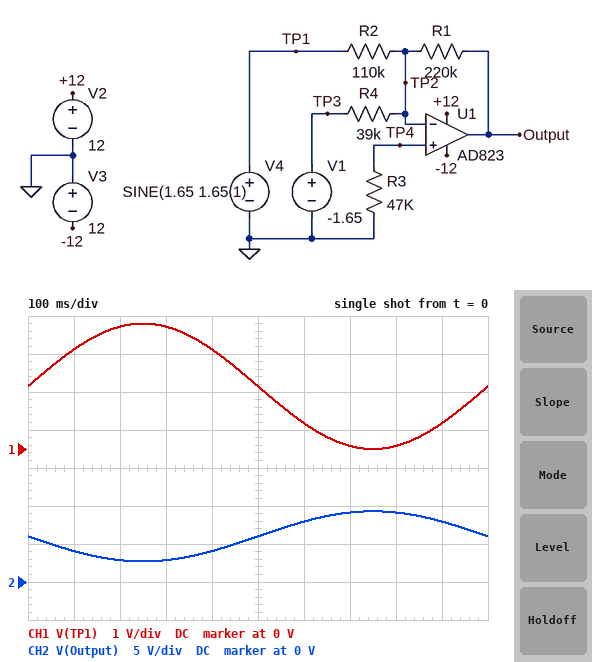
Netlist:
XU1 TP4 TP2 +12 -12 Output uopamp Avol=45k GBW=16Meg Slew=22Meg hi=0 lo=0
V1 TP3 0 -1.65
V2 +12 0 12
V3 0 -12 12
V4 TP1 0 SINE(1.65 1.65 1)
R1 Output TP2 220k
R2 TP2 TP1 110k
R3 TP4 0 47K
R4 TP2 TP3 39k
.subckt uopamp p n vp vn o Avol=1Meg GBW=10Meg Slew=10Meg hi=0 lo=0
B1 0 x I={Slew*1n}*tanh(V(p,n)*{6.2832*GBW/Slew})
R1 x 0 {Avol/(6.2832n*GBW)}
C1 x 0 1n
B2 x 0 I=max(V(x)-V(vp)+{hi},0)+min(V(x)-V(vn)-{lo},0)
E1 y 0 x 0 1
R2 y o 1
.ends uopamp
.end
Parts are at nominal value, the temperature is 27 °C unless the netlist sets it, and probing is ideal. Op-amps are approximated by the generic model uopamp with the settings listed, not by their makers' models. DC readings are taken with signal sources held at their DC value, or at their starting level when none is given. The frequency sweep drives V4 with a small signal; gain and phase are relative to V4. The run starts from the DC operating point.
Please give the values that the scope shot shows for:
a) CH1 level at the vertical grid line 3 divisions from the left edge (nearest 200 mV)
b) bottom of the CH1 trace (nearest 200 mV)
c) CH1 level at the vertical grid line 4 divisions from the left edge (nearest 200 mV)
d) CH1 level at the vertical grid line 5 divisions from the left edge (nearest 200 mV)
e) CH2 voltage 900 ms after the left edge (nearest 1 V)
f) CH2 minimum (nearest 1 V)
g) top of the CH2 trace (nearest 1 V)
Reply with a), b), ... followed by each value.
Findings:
a) 3.2 V
b) 0 V
c) 2.6 V
d) 1.6 V
e) 8 V
f) 3 V
g) 9 V
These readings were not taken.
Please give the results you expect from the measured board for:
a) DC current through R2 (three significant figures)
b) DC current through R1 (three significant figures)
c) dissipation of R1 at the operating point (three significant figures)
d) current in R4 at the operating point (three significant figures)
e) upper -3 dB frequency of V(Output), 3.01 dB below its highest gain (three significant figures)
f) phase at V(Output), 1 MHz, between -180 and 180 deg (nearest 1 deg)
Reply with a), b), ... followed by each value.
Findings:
a) 15.0 µA
b) 27.3 µA
c) 164 µW
d) 42.3 µA
e) 1.85 MHz
f) 152 deg
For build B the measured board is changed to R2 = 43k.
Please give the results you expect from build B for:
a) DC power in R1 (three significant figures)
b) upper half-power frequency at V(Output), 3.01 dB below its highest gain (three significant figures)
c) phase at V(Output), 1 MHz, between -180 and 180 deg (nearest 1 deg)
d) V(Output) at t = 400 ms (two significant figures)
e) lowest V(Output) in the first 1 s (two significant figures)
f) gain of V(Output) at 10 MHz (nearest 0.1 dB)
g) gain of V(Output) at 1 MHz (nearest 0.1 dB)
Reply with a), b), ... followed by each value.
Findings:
a) 3.41 µW
b) 1.36 MHz
c) 144 deg
d) -4.1 V
e) -7.6 V
f) -3.2 dB
g) 12.3 dB
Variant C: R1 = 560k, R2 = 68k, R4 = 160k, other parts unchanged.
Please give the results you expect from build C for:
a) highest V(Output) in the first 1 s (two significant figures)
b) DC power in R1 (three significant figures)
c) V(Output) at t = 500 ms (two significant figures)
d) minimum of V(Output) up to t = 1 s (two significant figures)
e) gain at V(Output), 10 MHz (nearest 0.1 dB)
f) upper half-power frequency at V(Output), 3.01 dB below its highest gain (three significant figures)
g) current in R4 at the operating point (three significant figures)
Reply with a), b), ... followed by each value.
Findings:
a) 5.8 V
b) 109 µW
c) -7.8 V
d) -12 V
e) 0.2 dB
f) 1.26 MHz
g) 10.3 µA
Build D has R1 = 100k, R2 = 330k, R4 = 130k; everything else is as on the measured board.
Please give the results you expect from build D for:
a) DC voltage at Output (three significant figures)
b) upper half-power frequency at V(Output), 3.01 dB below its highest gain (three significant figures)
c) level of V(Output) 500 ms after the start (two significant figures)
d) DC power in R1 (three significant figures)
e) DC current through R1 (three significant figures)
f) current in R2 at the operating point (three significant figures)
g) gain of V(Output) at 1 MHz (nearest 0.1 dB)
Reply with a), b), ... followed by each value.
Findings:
a) 769 mV
b) 7.72 MHz
c) 770 mV
d) 5.92 µW
e) 7.69 µA
f) 5.00 µA
g) -10.4 dB
